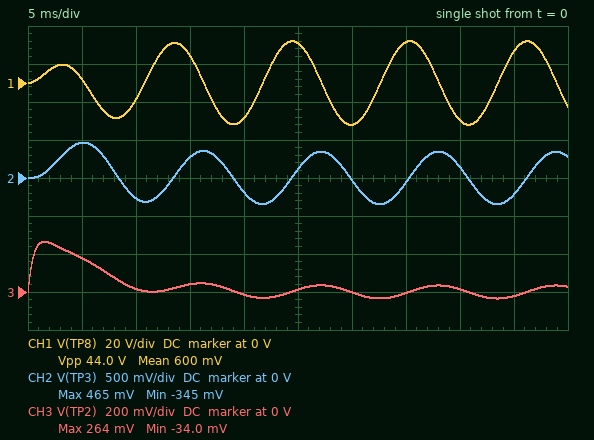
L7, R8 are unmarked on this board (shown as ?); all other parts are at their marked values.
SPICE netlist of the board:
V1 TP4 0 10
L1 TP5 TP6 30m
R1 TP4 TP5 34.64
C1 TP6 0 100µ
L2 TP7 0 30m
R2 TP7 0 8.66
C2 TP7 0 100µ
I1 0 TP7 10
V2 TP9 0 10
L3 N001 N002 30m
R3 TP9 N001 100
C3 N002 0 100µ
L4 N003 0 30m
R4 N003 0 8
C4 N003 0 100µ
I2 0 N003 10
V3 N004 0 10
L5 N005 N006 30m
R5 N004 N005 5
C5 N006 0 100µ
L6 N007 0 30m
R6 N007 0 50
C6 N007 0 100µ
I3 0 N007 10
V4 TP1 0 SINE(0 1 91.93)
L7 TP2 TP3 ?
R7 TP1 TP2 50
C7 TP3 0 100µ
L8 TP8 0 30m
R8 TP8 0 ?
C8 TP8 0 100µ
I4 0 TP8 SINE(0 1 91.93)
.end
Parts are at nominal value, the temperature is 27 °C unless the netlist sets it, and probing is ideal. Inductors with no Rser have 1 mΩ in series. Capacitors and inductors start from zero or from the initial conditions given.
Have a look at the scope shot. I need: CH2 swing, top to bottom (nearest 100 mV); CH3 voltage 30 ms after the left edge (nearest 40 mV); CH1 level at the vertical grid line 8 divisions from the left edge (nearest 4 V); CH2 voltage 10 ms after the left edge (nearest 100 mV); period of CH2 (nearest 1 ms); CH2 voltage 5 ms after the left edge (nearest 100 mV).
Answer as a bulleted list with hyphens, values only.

- 800 mV
- 0 V
- -20 V
- -300 mV
- 11 ms
- 500 mV
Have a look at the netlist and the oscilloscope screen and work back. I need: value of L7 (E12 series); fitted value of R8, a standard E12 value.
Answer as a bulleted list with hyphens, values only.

- 27 mH
- 22 Ω
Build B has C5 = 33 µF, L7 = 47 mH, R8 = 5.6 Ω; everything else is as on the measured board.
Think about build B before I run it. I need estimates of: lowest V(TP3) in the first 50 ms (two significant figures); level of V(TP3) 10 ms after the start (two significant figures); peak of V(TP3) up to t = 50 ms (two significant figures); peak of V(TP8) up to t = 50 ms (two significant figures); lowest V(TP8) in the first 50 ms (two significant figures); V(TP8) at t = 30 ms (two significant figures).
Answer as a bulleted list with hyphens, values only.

- -340 mV
- -220 mV
- 460 mV
- 5.6 V
- -6.0 V
- -5.6 V
